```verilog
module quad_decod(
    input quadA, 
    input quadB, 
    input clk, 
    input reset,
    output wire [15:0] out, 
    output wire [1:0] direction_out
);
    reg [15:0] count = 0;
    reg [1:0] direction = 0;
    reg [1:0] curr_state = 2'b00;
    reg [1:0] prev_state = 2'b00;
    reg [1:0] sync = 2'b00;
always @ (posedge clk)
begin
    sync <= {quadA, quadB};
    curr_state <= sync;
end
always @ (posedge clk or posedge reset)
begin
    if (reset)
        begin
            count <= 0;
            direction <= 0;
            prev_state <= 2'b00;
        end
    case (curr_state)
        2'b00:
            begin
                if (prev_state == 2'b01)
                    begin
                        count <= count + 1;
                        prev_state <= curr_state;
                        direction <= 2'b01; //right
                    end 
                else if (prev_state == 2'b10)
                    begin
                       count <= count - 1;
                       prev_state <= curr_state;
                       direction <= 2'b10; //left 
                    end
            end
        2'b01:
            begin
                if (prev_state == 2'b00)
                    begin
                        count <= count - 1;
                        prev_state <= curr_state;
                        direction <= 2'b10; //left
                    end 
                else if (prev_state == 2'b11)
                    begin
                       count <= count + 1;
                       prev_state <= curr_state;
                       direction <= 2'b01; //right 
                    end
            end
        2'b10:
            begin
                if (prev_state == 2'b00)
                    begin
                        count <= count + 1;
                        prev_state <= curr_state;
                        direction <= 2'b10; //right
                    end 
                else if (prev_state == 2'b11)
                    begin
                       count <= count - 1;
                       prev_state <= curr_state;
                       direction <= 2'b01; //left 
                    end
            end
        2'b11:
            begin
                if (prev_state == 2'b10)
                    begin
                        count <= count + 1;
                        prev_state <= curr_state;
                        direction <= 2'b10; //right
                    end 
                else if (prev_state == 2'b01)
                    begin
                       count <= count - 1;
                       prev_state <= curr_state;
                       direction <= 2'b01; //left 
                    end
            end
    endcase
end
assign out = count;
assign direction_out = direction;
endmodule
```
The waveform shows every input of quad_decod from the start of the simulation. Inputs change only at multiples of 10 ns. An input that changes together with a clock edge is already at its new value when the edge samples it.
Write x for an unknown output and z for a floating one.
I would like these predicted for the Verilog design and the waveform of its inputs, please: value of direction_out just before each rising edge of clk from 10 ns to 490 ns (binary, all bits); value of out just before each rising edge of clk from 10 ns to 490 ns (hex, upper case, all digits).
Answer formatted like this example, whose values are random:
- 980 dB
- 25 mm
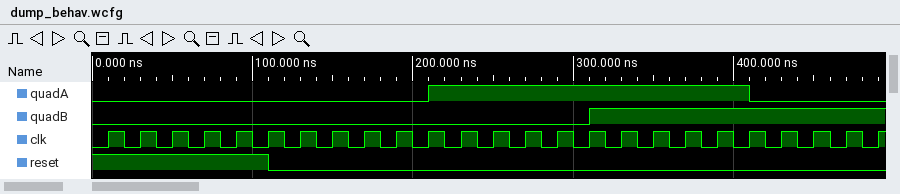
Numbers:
- 00, 00, 00, 00, 00, 00, 00, 00, 00, 00, 00, 00, 00, 10, 10, 10, 10, 10, 10, 10, 10, 10, 10, 01, 01
- 0000, 0000, 0000, 0000, 0000, 0000, 0000, 0000, 0000, 0000, 0000, 0000, 0000, 0001, 0001, 0001, 0001, 0001, 0002, 0002, 0002, 0002, 0002, 0003, 0003
